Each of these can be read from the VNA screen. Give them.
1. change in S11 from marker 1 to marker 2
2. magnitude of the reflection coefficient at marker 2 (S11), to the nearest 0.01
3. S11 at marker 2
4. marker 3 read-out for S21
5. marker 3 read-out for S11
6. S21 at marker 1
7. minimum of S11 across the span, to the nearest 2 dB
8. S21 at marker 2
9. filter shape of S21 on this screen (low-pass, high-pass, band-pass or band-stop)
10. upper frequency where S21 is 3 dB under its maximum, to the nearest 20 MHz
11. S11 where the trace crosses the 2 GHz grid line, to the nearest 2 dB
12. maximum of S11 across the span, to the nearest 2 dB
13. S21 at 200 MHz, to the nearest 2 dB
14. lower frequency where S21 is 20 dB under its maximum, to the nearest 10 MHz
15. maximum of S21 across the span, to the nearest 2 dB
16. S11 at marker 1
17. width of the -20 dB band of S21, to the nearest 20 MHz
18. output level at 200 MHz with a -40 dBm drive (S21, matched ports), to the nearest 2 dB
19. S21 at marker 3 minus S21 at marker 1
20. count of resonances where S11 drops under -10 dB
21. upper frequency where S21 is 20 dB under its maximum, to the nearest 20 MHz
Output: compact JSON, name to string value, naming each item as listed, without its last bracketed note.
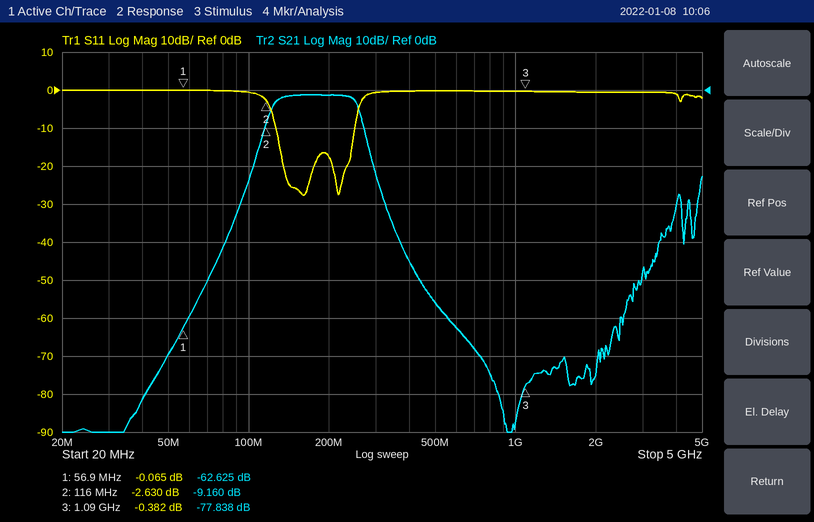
{"change in S11 from marker 1 to marker 2": "-2.565 dB", "magnitude of the reflection coefficient at marker 2 (S11), to the nearest 0.01": "0.74", "S11 at marker 2": "-2.630 dB", "marker 3 read-out for S21": "-77.838 dB", "marker 3 read-out for S11": "-0.382 dB", "S21 at marker 1": "-62.625 dB", "minimum of S11 across the span, to the nearest 2 dB": "-28 dB", "S21 at marker 2": "-9.160 dB", "filter shape of S21 on this screen": "band-pass", "upper frequency where S21 is 3 dB under its maximum, to the nearest 20 MHz": "260 MHz", "S11 where the trace crosses the 2 GHz grid line, to the nearest 2 dB": "0 dB", "maximum of S11 across the span, to the nearest 2 dB": "0 dB", "S21 at 200 MHz, to the nearest 2 dB": "-2 dB", "lower frequency where S21 is 20 dB under its maximum, to the nearest 10 MHz": "100 MHz", "maximum of S21 across the span, to the nearest 2 dB": "-2 dB", "S11 at marker 1": "-0.065 dB", "width of the -20 dB band of S21, to the nearest 20 MHz": "200 MHz", "output level at 200 MHz with a -40 dBm drive (S21, matched ports), to the nearest 2 dB": "-42 dBm", "S21 at marker 3 minus S21 at marker 1": "-15.213 dB", "count of resonances where S11 drops under -10 dB": "2", "upper frequency where S21 is 20 dB under its maximum, to the nearest 20 MHz": "300 MHz"}
